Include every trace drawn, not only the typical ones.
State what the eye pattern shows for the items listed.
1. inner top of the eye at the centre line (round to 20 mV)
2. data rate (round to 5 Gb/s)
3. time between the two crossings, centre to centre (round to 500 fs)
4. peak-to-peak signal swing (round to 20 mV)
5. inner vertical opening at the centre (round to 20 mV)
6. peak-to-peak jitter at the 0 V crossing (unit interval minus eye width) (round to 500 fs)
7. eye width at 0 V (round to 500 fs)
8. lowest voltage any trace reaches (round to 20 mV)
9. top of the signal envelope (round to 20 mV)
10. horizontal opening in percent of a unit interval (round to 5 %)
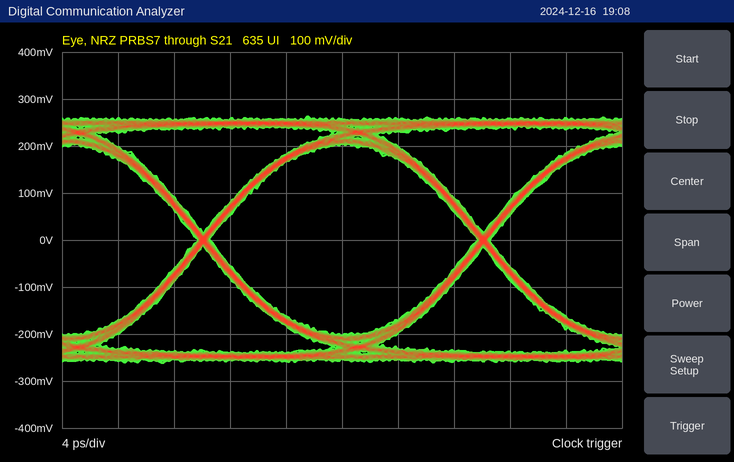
200 mV
50 Gb/s
20.0 ps
520 mV
400 mV
1.0 ps
19.0 ps
-260 mV
260 mV
95 %
